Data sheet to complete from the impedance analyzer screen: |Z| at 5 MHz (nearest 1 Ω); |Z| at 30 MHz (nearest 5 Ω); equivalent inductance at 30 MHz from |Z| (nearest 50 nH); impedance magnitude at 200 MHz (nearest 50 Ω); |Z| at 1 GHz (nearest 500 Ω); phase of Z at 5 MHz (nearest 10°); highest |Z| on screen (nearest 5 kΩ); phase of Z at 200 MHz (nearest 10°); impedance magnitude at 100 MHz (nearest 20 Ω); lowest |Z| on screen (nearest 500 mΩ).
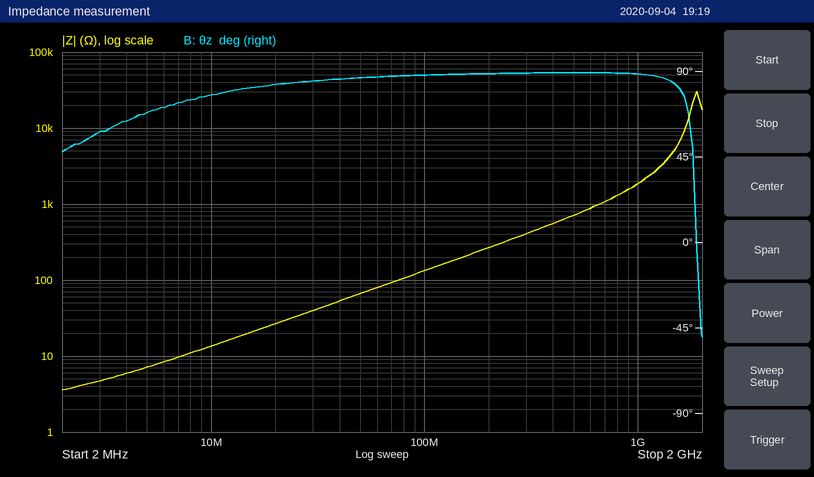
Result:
7 Ω
40 Ω
200 nH
250 Ω
2.0 kΩ
70°
30 kΩ
90°
140 Ω
3.5 Ω
